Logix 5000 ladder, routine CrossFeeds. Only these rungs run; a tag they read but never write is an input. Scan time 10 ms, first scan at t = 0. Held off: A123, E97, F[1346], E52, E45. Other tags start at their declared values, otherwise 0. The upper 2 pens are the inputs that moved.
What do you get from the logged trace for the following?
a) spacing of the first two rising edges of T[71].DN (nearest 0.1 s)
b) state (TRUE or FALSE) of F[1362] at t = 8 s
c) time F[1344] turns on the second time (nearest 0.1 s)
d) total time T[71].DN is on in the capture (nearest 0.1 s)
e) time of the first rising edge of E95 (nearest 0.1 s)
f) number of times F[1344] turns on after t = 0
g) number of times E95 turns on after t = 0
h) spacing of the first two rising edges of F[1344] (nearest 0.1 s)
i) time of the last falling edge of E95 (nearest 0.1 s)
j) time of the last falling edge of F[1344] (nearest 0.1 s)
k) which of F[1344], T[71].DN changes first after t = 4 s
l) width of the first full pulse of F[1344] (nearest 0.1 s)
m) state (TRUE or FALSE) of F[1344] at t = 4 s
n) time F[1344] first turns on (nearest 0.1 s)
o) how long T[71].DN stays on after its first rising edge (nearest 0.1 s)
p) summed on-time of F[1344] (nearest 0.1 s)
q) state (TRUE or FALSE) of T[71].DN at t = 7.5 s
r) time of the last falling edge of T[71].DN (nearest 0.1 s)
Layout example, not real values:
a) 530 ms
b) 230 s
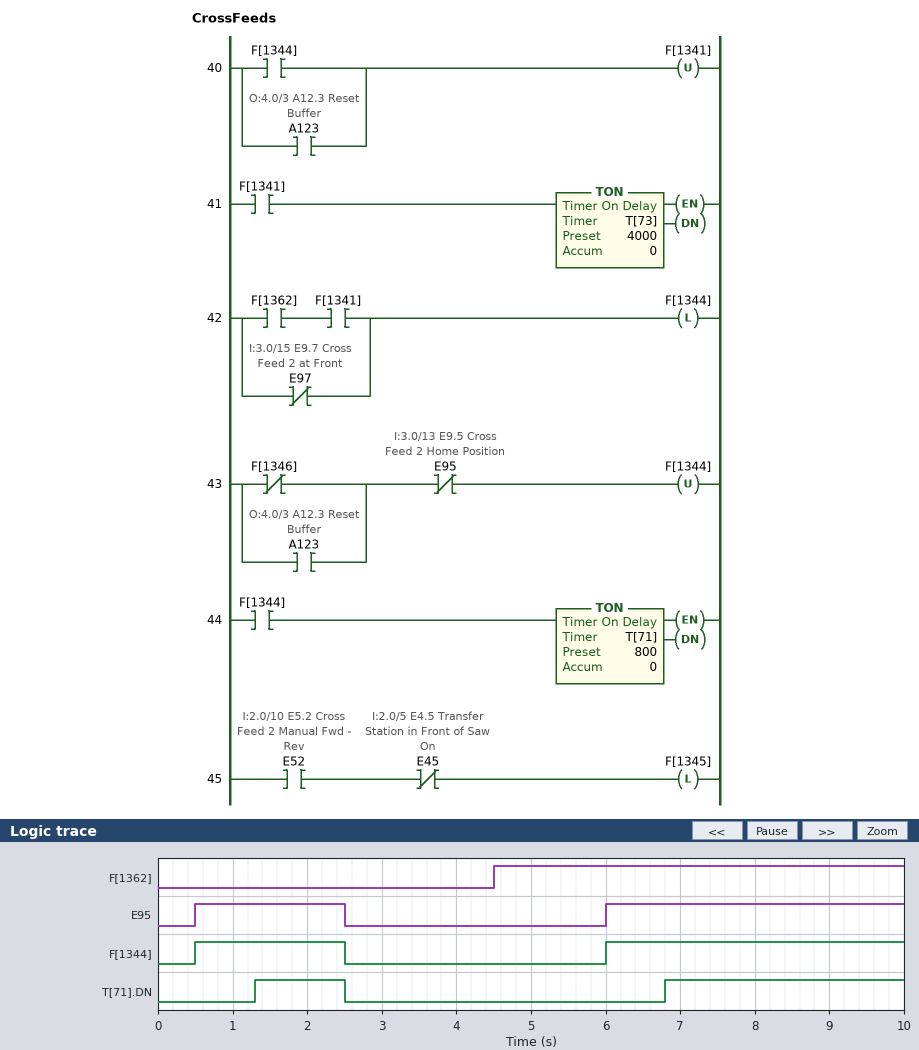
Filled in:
a) 5.5 s
b) TRUE
c) 6.0 s
d) 4.4 s
e) 0.5 s
f) 2
g) 2
h) 5.5 s
i) 2.5 s
j) 2.5 s
k) F[1344]
l) 2.0 s
m) FALSE
n) 0.5 s
o) 1.2 s
p) 6.0 s
q) TRUE
r) 2.5 s
